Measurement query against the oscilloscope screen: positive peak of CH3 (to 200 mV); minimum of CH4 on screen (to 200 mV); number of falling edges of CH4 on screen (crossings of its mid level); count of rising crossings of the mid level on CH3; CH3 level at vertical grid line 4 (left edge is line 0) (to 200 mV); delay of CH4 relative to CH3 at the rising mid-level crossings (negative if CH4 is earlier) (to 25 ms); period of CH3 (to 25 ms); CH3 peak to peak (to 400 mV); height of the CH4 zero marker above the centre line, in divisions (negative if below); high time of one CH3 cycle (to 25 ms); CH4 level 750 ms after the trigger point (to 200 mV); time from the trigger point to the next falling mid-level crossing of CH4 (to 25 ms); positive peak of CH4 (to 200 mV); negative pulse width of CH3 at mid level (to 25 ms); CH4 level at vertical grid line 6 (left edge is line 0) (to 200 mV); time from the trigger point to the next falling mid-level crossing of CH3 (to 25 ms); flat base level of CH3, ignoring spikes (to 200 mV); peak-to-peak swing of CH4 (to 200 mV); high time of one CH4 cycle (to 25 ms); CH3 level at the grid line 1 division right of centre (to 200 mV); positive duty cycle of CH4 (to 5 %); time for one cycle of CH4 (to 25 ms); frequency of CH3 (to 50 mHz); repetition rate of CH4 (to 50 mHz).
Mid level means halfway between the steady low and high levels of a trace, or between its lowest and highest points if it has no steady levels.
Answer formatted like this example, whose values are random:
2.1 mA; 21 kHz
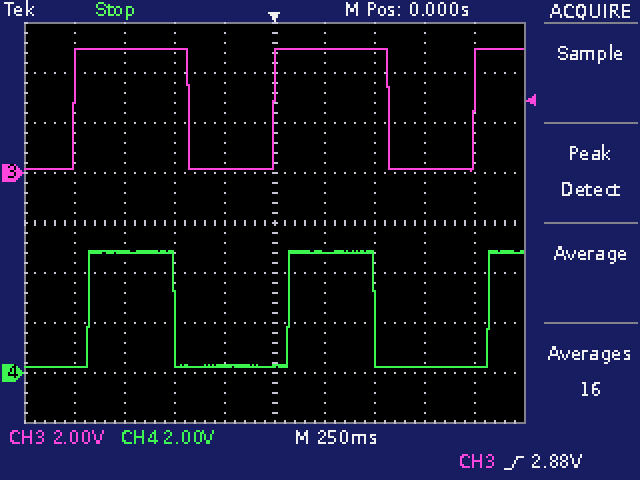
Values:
5.0 V; 200 mV; 2; 3; 200 mV; +75 ms; 1.000 s; 4.8 V; -3.0 div; 575 ms; 200 mV; 500 ms; 4.8 V; 425 ms; 4.8 V; 575 ms; 200 mV; 4.6 V; 425 ms; 5.0 V; 45 %; 1.000 s; 1.00 Hz; 1.00 Hz
